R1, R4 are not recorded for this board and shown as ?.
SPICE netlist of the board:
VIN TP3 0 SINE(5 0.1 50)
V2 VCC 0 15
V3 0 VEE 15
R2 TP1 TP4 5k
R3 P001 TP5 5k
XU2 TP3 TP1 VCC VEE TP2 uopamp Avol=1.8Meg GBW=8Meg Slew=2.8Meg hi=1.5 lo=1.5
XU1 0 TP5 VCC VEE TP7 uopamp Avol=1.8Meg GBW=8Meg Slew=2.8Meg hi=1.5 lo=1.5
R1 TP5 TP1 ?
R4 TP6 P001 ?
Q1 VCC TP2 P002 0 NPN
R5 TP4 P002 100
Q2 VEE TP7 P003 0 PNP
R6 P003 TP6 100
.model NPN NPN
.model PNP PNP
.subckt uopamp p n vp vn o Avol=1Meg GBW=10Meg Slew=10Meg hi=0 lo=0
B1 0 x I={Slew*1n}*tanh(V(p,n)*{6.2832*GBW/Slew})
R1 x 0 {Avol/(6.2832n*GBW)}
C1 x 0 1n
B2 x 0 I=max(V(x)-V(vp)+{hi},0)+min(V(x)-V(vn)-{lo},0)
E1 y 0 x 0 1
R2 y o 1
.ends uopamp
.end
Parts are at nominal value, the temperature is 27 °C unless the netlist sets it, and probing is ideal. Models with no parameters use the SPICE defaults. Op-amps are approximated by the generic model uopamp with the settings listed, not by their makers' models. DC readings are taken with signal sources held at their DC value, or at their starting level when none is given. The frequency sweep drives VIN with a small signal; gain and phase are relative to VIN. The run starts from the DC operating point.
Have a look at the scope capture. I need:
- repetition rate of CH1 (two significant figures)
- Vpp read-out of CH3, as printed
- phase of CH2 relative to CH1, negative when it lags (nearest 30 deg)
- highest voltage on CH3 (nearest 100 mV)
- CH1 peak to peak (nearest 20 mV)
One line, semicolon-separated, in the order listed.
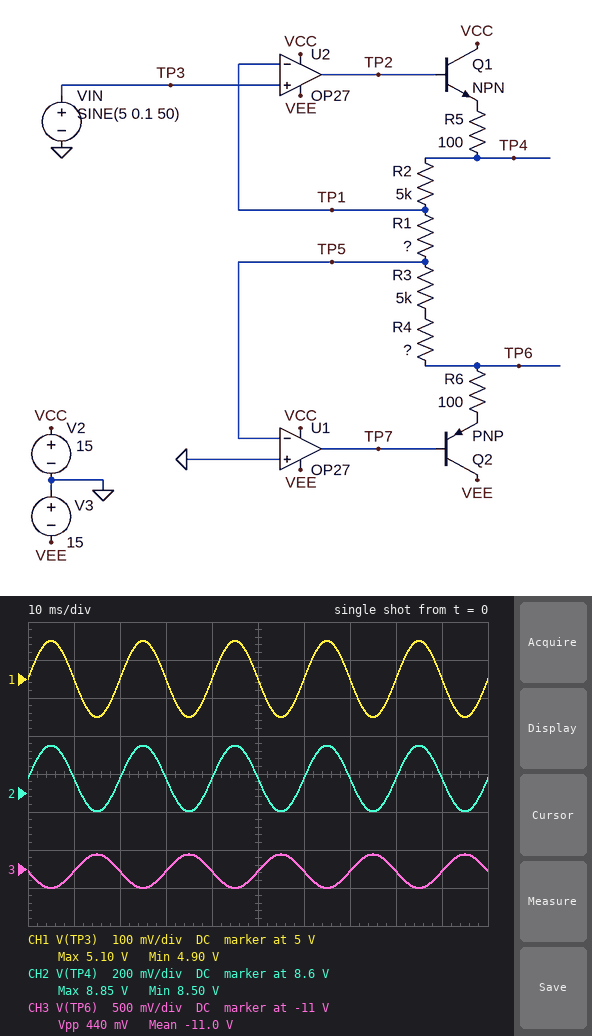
50 Hz; 440 mV; 0 deg; -10.8 V; 200 mV
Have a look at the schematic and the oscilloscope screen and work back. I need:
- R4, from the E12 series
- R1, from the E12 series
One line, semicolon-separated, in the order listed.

10 kΩ; 6.8 kΩ
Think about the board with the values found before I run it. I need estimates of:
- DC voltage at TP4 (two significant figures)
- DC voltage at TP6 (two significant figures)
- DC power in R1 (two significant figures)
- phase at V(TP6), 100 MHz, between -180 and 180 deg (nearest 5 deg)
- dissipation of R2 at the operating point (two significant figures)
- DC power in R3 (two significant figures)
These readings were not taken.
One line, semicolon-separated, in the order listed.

8.7 V; -11 V; 3.7 mW; 0 deg; 2.7 mW; 2.7 mW
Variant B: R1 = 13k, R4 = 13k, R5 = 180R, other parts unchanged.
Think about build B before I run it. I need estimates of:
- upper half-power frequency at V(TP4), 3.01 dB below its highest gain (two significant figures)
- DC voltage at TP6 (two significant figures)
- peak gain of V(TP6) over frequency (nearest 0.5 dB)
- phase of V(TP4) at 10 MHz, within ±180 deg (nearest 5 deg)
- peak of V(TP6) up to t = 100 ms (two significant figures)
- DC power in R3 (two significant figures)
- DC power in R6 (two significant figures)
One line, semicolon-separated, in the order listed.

4.5 MHz; -6.9 V; 3.0 dB; -55 deg; -6.8 V; 740 µW; 15 µW
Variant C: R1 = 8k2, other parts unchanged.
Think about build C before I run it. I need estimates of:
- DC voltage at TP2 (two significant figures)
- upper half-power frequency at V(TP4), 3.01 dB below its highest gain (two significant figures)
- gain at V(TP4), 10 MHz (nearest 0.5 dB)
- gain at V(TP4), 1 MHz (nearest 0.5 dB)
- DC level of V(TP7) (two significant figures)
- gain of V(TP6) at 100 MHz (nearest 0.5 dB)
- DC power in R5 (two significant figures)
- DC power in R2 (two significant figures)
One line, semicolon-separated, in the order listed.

8.9 V; 3.3 MHz; -4.0 dB; 3.5 dB; -10 V; -49.5 dB; 37 µW; 1.9 mW
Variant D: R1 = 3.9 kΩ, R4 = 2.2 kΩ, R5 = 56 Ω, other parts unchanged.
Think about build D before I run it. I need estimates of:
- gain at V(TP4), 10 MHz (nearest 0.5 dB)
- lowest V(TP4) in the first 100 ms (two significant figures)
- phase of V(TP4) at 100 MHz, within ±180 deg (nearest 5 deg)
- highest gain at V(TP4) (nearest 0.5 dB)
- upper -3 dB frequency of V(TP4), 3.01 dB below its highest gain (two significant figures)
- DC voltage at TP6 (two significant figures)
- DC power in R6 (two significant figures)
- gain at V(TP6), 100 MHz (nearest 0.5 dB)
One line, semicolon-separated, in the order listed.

-3.5 dB; 11 V; -85 deg; 7.0 dB; 2.2 MHz; -9.2 V; 160 µW; -51.0 dB
